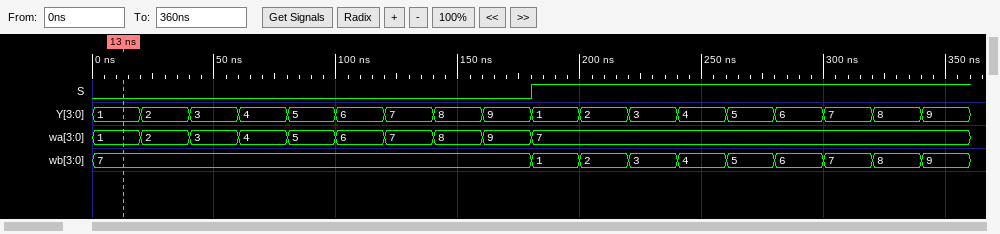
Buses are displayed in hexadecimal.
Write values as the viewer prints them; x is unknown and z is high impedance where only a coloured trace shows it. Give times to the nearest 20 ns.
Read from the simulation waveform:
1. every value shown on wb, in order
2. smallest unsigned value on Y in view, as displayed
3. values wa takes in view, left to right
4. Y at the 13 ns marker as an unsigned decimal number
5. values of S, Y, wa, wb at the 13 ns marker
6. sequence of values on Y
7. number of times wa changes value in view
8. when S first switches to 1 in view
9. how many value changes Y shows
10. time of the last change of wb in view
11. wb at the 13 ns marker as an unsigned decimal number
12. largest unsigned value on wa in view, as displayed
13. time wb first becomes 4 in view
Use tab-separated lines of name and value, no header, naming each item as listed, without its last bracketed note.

every value shown on wb, in order	7, 1, 2, 3, 4, 5, 6, 7, 8, 9
smallest unsigned value on Y in view, as displayed	1
values wa takes in view, left to right	1, 2, 3, 4, 5, 6, 7, 8, 9, 7
Y at the 13 ns marker as an unsigned decimal number	1
values of S, Y, wa, wb at the 13 ns marker	S=0, Y=1, wa=1, wb=7
sequence of values on Y	1, 2, 3, 4, 5, 6, 7, 8, 9, 1, 2, 3, 4, 5, 6, 7, 8, 9
number of times wa changes value in view	9
when S first switches to 1 in view	180 ns
how many value changes Y shows	17
time of the last change of wb in view	340 ns
wb at the 13 ns marker as an unsigned decimal number	7
largest unsigned value on wa in view, as displayed	9
time wb first becomes 4 in view	240 ns
